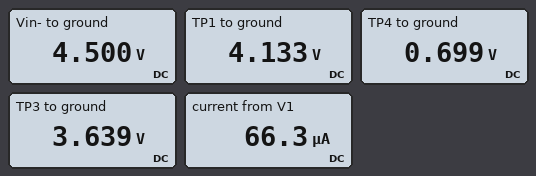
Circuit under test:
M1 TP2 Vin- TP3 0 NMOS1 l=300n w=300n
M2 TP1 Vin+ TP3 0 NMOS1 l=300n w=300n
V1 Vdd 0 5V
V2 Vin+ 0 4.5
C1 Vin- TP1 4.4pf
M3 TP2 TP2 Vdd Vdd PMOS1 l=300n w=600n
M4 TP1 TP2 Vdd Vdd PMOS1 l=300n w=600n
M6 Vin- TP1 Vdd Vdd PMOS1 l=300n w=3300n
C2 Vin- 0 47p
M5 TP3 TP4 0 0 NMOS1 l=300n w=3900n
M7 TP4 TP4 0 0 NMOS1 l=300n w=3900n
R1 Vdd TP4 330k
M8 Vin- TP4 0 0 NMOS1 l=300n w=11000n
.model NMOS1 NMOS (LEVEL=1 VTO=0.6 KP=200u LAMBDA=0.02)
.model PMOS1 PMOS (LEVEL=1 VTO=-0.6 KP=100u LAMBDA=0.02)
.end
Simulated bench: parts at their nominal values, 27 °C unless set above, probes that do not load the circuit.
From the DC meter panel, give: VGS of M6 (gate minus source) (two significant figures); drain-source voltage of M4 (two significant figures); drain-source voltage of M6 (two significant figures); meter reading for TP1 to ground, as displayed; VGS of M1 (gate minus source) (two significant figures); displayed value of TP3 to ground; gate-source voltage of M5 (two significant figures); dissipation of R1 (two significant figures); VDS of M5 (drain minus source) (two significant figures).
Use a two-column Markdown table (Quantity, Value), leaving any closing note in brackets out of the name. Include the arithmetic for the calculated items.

| Quantity | Value |
|---|---|
| VGS of M6 (gate minus source) | 4.133 V - 5 V = -870 mV |
| drain-source voltage of M4 | 4.133 V - 5 V = -870 mV |
| drain-source voltage of M6 | 4.5 V - 5 V = -500 mV |
| meter reading for TP1 to ground, as displayed | 4.133 V |
| VGS of M1 (gate minus source) | 4.5 V - 3.639 V = 860 mV |
| displayed value of TP3 to ground | 3.639 V |
| gate-source voltage of M5 | 699 mV = 700 mV |
| dissipation of R1 | (5 V - 699 mV)^2 / 330 kΩ = 56 µW |
| VDS of M5 (drain minus source) | 3.639 V = 3.6 V |
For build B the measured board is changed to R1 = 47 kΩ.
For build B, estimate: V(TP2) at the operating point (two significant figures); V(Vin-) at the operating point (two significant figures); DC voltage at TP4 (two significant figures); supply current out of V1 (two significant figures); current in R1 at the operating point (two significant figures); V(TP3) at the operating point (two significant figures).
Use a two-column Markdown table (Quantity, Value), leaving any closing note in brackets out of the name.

| Quantity | Value |
|---|---|
| V(TP2) at the operating point | 3.7 V |
| V(Vin-) at the operating point | 4.5 V |
| DC voltage at TP4 | 860 mV |
| supply current out of V1 | 450 µA |
| current in R1 at the operating point | 88 µA |
| V(TP3) at the operating point | 3.2 V |
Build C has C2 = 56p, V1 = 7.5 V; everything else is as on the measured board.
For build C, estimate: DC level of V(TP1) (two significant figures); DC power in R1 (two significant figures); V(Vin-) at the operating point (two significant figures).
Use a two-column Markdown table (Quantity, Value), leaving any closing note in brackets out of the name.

| Quantity | Value |
|---|---|
| DC level of V(TP1) | 6.6 V |
| DC power in R1 | 140 µW |
| V(Vin-) at the operating point | 4.5 V |
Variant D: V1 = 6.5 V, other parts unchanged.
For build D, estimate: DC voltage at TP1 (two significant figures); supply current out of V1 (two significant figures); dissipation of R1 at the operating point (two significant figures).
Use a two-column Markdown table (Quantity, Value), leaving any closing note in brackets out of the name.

| Quantity | Value |
|---|---|
| DC voltage at TP1 | 5.6 V |
| supply current out of V1 | 89 µA |
| dissipation of R1 at the operating point | 100 µW |
